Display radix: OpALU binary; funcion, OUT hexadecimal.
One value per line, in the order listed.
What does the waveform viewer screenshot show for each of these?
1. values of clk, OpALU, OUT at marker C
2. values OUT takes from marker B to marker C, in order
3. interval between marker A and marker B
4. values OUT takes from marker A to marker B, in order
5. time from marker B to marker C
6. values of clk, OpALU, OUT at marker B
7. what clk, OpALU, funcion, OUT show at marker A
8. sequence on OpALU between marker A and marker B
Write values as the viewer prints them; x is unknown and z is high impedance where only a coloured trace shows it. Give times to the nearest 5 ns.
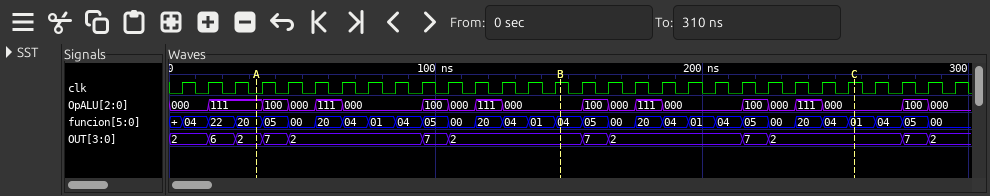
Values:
clk=1, OpALU=000, OUT=2
2, 7, 2, 7, 2
115 ns
2, 7, 2, 7, 2
110 ns
clk=1, OpALU=000, OUT=2
clk=0, OpALU=111, funcion=20, OUT=2
111, 100, 000, 111, 000, 100, 000, 111, 000
